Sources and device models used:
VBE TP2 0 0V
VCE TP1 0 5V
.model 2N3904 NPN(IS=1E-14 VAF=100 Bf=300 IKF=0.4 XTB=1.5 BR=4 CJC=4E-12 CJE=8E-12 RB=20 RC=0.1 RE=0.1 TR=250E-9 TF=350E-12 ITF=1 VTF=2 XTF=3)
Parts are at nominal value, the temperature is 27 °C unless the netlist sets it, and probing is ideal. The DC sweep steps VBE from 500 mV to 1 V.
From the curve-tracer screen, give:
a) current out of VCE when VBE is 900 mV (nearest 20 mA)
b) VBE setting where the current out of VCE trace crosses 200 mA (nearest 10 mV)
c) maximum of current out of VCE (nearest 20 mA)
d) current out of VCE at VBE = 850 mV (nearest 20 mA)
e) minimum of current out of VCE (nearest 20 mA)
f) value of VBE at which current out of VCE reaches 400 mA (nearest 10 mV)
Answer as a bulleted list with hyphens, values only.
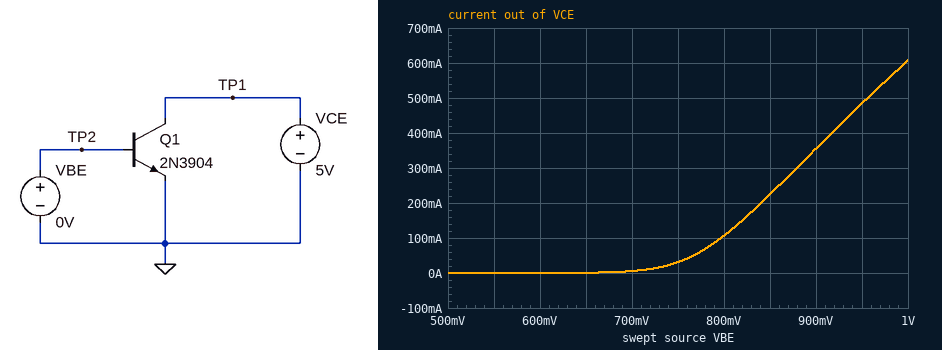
- 360 mA
- 840 mV
- 600 mA
- 220 mA
- 0 A
- 920 mV
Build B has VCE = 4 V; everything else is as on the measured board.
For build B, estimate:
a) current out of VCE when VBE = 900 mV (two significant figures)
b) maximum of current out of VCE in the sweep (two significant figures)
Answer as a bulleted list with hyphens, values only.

- 350 mA
- 600 mA
